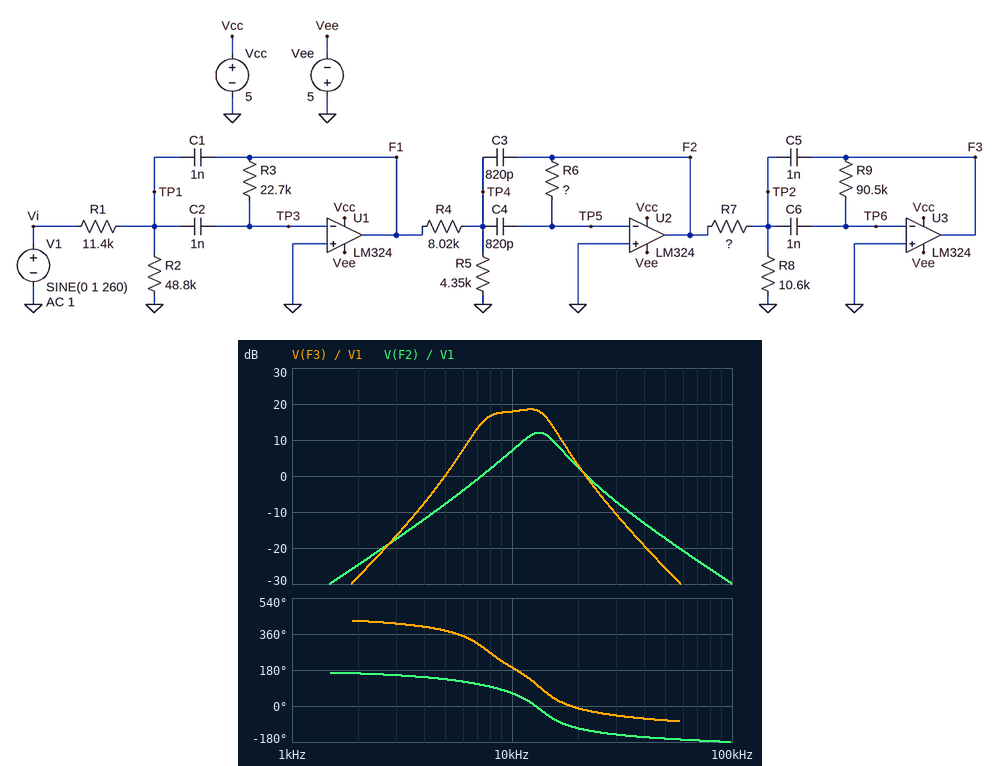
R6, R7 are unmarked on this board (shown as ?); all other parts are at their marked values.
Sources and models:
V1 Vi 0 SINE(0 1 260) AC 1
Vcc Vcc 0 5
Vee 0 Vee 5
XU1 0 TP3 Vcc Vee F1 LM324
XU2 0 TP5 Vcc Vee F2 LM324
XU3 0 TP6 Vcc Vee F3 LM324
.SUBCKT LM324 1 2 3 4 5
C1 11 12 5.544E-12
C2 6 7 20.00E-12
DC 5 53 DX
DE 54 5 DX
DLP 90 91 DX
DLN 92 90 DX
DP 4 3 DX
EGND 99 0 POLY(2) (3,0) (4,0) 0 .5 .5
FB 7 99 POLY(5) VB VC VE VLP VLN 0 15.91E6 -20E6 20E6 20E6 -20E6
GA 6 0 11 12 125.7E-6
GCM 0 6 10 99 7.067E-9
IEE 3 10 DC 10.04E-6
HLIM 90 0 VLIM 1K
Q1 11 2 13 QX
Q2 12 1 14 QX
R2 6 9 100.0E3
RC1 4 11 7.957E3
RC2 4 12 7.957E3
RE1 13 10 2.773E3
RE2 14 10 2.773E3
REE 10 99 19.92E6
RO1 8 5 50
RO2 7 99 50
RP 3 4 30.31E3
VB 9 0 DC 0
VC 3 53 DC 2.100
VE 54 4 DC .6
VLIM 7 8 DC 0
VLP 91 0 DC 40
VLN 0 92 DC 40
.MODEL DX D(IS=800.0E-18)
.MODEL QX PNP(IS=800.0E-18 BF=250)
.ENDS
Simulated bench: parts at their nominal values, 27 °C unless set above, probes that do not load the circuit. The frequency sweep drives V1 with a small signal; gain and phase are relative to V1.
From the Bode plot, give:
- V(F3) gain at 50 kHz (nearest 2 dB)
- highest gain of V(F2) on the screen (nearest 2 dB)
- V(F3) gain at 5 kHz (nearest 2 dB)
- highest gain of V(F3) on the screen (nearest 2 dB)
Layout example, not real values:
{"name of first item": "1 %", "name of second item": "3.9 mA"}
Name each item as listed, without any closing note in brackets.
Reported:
{"V(F3) gain at 50 kHz": "-26 dB", "highest gain of V(F2) on the screen": "12 dB", "V(F3) gain at 5 kHz": "0 dB", "highest gain of V(F3) on the screen": "18 dB"}
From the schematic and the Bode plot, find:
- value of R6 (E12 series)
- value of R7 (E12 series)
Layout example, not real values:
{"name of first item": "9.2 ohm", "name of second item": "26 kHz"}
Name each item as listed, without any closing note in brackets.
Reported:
{"value of R6": "68 kΩ", "value of R7": "8.2 kΩ"}
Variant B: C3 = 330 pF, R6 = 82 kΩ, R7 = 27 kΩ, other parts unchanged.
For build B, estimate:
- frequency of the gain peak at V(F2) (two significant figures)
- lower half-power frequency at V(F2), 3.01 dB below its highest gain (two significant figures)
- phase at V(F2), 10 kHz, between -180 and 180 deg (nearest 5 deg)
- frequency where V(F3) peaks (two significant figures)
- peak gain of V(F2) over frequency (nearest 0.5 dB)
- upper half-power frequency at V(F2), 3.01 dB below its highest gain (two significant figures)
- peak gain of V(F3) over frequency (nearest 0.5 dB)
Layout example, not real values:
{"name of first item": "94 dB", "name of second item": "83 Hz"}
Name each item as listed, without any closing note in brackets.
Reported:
{"frequency of the gain peak at V(F2)": "18 kHz", "lower half-power frequency at V(F2), 3.01 dB below its highest gain": "14 kHz", "phase at V(F2), 10 kHz, between -180 and 180 deg": "80 deg", "frequency where V(F3) peaks": "17 kHz", "peak gain of V(F2) over frequency": "15.0 dB", "upper half-power frequency at V(F2), 3.01 dB below its highest gain": "21 kHz", "peak gain of V(F3) over frequency": "6.0 dB"}
